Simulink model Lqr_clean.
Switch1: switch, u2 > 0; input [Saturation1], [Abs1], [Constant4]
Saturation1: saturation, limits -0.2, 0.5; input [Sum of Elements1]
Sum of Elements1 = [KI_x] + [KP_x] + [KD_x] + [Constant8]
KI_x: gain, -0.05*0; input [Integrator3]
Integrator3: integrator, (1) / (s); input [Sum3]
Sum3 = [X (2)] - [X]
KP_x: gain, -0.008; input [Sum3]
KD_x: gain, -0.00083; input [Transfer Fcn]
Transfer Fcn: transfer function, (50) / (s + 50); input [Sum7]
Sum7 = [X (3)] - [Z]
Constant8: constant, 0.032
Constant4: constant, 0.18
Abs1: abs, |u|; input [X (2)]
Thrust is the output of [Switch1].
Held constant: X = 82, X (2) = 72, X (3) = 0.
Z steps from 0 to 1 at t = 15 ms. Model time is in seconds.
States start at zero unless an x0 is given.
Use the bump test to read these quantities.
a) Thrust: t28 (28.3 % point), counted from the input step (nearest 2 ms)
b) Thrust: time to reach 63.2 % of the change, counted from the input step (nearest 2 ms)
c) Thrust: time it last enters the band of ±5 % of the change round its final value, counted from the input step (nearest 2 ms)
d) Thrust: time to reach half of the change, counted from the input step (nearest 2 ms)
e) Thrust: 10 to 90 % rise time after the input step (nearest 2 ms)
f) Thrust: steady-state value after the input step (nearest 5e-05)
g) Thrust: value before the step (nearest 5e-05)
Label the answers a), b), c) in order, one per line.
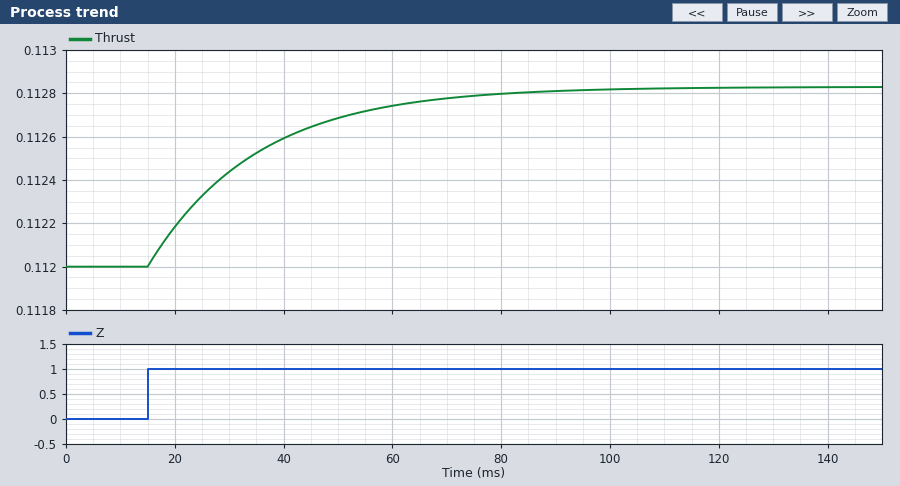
a) 6 ms
b) 20 ms
c) 60 ms
d) 14 ms
e) 44 ms
f) 0.11285
g) 0.11200
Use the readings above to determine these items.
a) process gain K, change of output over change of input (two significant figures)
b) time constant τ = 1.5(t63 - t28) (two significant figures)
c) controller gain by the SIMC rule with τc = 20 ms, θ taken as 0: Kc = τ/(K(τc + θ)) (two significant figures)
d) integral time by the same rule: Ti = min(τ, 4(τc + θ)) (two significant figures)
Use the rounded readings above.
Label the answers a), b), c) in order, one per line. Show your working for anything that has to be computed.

a) (0.11285 - 0.112) / 1 = 0.00085
b) 1.5 × (20 - 6) = 21 ms
c) 21 / (0.00085 × (20 + 0)) = 1200
d) min(21, 4 × (20 + 0)) = 21 ms
